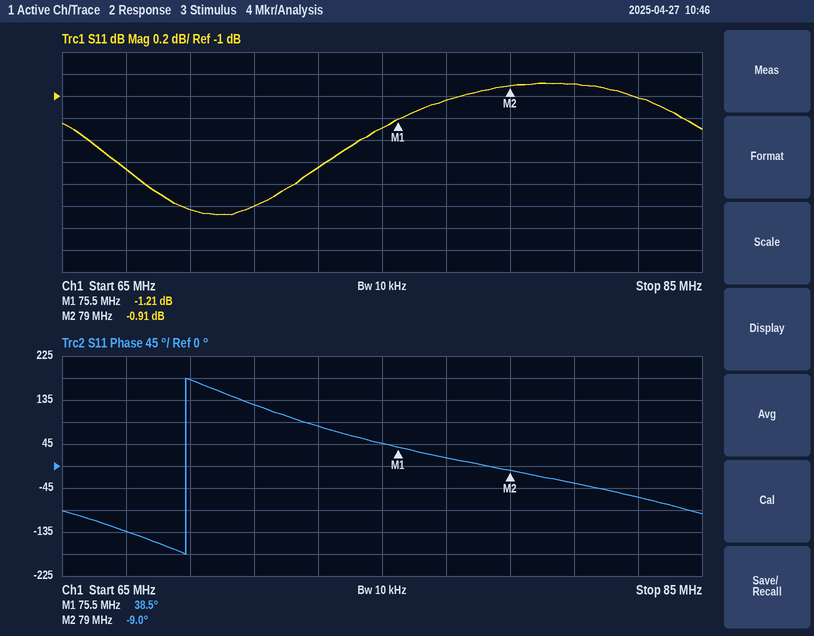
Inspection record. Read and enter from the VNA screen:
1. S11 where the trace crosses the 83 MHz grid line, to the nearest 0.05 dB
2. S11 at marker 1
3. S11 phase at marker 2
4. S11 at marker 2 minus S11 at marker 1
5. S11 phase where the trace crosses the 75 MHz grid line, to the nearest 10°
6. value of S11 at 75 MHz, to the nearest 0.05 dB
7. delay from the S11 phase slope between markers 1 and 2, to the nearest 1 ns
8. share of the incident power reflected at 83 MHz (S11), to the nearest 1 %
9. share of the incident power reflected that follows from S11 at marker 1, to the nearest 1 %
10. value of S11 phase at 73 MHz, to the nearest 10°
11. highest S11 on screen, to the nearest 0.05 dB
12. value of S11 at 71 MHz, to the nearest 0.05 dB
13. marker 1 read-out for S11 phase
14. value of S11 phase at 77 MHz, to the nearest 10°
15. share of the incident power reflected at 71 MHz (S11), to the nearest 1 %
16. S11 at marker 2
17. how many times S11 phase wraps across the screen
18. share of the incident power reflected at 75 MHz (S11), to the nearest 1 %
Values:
-1.00 dB
-1.21 dB
-9.0°
0.30 dB
50°
-1.30 dB
38 ns
79 %
76 %
80°
-0.90 dB
-2.00 dB
38.5°
20°
63 %
-0.91 dB
1
74 %
